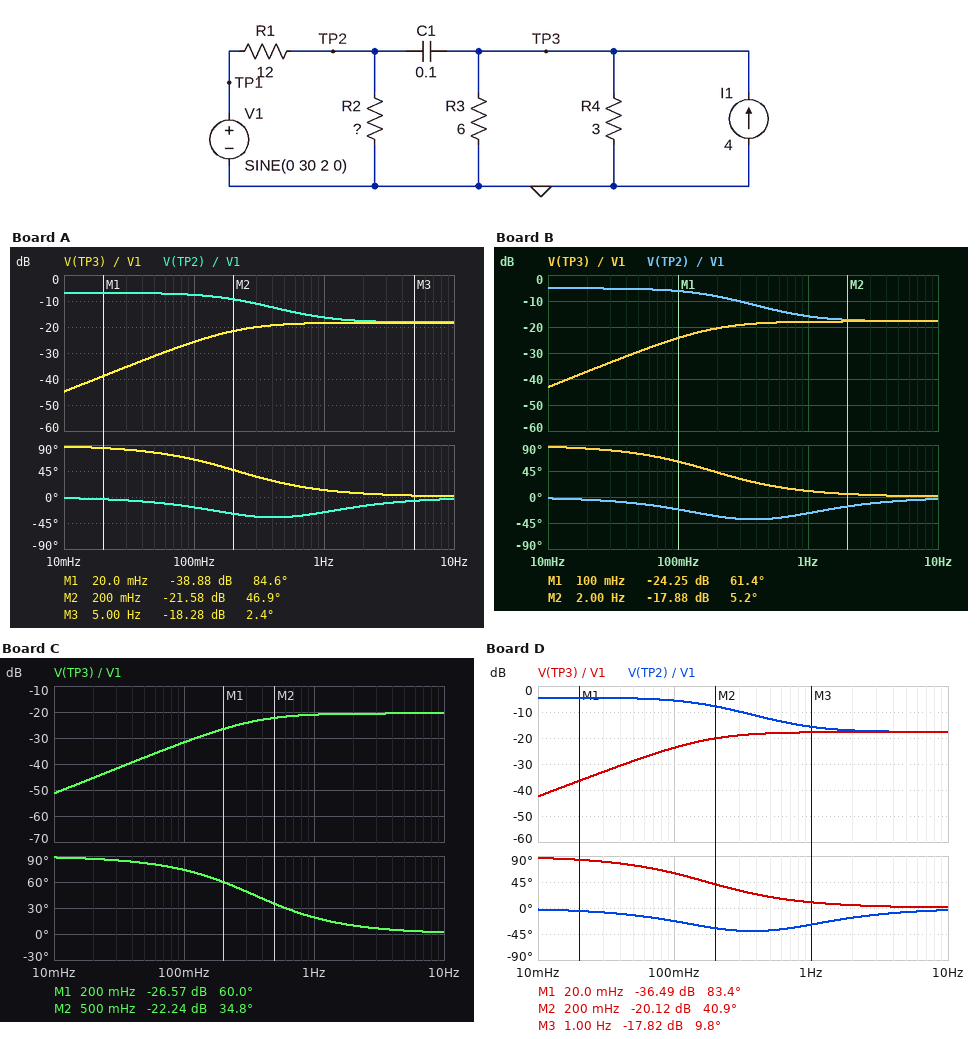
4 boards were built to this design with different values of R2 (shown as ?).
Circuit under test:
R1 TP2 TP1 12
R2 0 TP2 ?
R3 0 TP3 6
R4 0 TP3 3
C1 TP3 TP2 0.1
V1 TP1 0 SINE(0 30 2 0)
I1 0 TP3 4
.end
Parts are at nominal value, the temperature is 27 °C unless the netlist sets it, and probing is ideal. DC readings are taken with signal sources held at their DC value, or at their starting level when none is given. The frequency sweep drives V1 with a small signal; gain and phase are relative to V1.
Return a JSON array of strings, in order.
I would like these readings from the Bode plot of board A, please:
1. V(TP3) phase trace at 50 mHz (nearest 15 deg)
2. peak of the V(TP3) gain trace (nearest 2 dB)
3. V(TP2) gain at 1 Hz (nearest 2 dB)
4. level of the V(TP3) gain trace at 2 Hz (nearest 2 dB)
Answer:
["75 deg", "-18 dB", "-16 dB", "-18 dB"]
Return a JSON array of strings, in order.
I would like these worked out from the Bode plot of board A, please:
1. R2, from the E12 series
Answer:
["10 Ω"]
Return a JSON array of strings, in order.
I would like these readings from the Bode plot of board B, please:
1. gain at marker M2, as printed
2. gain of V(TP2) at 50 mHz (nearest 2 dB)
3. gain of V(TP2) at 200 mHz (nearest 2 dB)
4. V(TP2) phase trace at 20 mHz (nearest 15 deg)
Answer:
["-17.88 dB", "-6 dB", "-8 dB", "0 deg"]
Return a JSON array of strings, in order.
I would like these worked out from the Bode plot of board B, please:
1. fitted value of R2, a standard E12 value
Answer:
["15 Ω"]
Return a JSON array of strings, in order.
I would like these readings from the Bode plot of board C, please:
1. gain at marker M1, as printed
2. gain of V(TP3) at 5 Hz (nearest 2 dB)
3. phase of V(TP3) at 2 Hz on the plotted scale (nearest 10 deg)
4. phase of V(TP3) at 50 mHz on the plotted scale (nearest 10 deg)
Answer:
["-26.57 dB", "-20 dB", "10 deg", "80 deg"]
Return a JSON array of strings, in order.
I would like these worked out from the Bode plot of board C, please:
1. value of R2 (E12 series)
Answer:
["3.3 Ω"]
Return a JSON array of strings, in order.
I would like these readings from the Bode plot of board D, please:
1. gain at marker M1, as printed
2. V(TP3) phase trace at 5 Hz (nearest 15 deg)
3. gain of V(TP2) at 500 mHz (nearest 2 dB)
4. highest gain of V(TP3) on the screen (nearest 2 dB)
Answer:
["-36.49 dB", "0 deg", "-12 dB", "-18 dB"]
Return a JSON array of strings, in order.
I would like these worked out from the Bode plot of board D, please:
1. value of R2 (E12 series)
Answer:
["18 Ω"]
